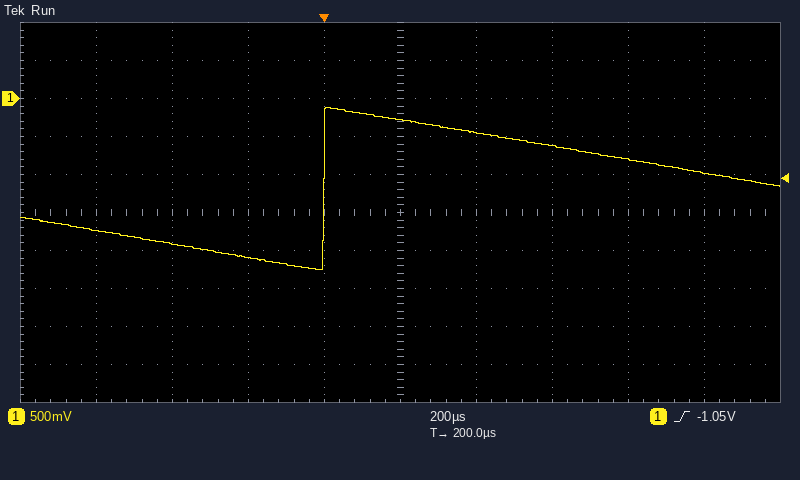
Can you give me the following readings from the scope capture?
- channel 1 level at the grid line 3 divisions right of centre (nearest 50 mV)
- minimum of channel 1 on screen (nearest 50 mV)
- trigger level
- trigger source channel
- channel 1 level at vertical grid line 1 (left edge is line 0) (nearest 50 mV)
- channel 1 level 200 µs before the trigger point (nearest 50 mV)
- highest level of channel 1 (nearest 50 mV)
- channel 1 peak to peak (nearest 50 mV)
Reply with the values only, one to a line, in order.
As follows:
-800 mV
-2.25 V
-1.05 V
channel 1
-1.75 V
-2.10 V
-100 mV
2.15 V
